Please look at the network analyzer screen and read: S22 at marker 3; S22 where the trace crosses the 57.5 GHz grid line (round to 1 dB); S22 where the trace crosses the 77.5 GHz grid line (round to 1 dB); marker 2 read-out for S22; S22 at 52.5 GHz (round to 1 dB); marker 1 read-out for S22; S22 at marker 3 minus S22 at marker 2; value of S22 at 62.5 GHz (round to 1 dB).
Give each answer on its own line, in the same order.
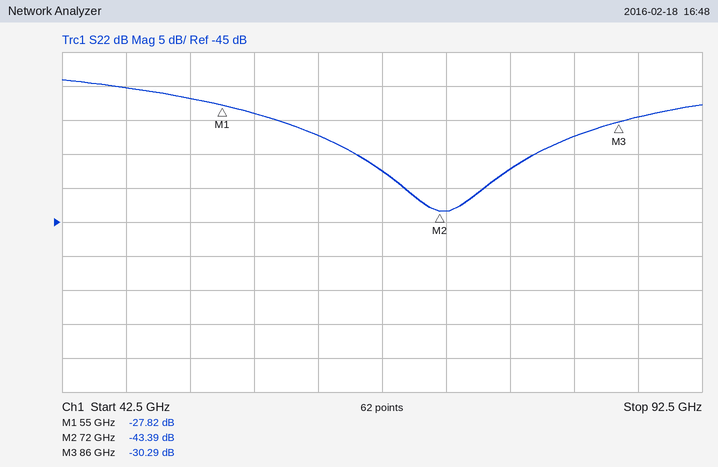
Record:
-30.29 dB
-29 dB
-37 dB
-43.39 dB
-27 dB
-27.82 dB
13.10 dB
-32 dB
